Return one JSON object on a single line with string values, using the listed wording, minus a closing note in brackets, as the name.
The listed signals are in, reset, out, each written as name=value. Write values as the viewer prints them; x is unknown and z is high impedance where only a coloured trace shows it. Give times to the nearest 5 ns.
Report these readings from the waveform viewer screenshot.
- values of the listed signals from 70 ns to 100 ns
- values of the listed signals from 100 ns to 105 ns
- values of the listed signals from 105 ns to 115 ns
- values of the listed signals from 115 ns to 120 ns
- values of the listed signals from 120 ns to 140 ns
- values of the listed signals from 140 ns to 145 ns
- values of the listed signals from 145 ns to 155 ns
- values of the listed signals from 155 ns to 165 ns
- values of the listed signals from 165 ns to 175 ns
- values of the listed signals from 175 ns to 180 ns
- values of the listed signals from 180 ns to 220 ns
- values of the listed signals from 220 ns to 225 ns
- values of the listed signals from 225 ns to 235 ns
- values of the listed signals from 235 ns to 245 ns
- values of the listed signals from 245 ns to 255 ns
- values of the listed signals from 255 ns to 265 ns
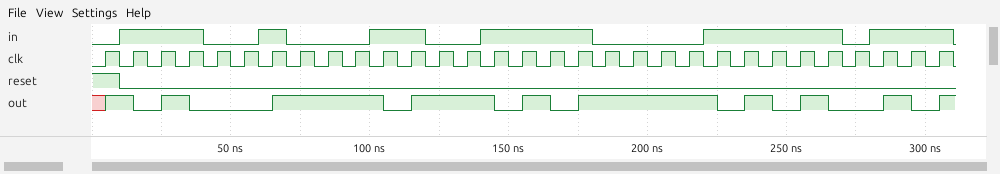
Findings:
{"values of the listed signals from 70 ns to 100 ns": "in=0, reset=0, out=1", "values of the listed signals from 100 ns to 105 ns": "in=1, reset=0, out=1", "values of the listed signals from 105 ns to 115 ns": "in=1, reset=0, out=0", "values of the listed signals from 115 ns to 120 ns": "in=1, reset=0, out=1", "values of the listed signals from 120 ns to 140 ns": "in=0, reset=0, out=1", "values of the listed signals from 140 ns to 145 ns": "in=1, reset=0, out=1", "values of the listed signals from 145 ns to 155 ns": "in=1, reset=0, out=0", "values of the listed signals from 155 ns to 165 ns": "in=1, reset=0, out=1", "values of the listed signals from 165 ns to 175 ns": "in=1, reset=0, out=0", "values of the listed signals from 175 ns to 180 ns": "in=1, reset=0, out=1", "values of the listed signals from 180 ns to 220 ns": "in=0, reset=0, out=1", "values of the listed signals from 220 ns to 225 ns": "in=1, reset=0, out=1", "values of the listed signals from 225 ns to 235 ns": "in=1, reset=0, out=0", "values of the listed signals from 235 ns to 245 ns": "in=1, reset=0, out=1", "values of the listed signals from 245 ns to 255 ns": "in=1, reset=0, out=0", "values of the listed signals from 255 ns to 265 ns": "in=1, reset=0, out=1"}
